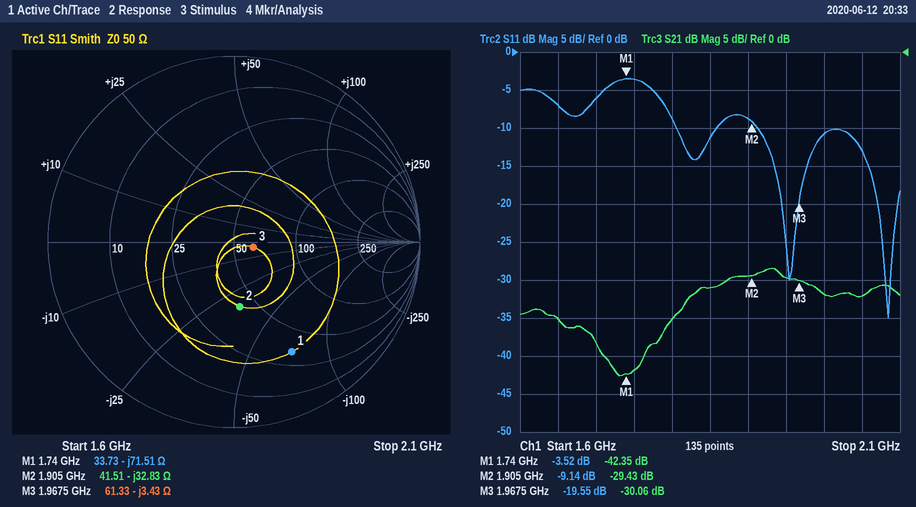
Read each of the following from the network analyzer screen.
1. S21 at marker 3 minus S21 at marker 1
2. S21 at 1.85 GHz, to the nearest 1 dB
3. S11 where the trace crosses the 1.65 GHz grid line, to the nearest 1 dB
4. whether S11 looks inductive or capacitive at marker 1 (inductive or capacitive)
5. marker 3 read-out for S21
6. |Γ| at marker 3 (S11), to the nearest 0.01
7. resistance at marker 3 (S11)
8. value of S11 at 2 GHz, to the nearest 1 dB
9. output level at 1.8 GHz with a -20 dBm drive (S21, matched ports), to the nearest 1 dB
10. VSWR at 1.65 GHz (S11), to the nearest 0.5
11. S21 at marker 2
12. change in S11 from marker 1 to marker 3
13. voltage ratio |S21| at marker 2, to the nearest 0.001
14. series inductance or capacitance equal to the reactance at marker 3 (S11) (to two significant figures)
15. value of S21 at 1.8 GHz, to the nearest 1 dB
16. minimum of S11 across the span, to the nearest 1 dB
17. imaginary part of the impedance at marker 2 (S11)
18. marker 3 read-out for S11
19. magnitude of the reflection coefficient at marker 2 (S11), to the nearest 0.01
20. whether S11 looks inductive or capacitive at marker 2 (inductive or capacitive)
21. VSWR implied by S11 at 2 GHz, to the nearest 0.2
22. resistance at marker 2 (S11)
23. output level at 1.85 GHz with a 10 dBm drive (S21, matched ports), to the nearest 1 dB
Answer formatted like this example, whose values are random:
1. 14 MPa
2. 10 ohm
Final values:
1. 12.29 dB
2. -31 dB
3. -7 dB
4. capacitive
5. -30.06 dB
6. 0.11
7. 61.33 Ω
8. -11 dB
9. -55 dBm
10. 2.5
11. -29.43 dB
12. -16.03 dB
13. 0.034
14. 24 pF
15. -35 dB
16. -35 dB
17. -32.83 Ω
18. -19.55 dB
19. 0.35
20. capacitive
21. 1.8
22. 41.51 Ω
23. -21 dBm
